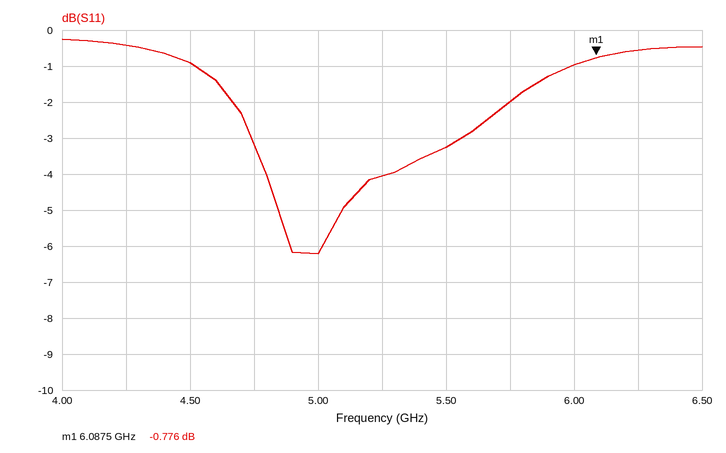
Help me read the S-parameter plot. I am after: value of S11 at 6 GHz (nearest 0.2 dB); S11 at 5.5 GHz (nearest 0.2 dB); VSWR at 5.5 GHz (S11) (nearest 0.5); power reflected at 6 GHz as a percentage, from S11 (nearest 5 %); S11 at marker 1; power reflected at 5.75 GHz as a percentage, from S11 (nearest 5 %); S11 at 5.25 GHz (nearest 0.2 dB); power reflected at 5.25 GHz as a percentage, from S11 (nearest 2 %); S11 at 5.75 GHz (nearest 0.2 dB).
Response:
-1.0 dB
-3.2 dB
5.5
80 %
-0.776 dB
65 %
-4.0 dB
40 %
-2.0 dB
